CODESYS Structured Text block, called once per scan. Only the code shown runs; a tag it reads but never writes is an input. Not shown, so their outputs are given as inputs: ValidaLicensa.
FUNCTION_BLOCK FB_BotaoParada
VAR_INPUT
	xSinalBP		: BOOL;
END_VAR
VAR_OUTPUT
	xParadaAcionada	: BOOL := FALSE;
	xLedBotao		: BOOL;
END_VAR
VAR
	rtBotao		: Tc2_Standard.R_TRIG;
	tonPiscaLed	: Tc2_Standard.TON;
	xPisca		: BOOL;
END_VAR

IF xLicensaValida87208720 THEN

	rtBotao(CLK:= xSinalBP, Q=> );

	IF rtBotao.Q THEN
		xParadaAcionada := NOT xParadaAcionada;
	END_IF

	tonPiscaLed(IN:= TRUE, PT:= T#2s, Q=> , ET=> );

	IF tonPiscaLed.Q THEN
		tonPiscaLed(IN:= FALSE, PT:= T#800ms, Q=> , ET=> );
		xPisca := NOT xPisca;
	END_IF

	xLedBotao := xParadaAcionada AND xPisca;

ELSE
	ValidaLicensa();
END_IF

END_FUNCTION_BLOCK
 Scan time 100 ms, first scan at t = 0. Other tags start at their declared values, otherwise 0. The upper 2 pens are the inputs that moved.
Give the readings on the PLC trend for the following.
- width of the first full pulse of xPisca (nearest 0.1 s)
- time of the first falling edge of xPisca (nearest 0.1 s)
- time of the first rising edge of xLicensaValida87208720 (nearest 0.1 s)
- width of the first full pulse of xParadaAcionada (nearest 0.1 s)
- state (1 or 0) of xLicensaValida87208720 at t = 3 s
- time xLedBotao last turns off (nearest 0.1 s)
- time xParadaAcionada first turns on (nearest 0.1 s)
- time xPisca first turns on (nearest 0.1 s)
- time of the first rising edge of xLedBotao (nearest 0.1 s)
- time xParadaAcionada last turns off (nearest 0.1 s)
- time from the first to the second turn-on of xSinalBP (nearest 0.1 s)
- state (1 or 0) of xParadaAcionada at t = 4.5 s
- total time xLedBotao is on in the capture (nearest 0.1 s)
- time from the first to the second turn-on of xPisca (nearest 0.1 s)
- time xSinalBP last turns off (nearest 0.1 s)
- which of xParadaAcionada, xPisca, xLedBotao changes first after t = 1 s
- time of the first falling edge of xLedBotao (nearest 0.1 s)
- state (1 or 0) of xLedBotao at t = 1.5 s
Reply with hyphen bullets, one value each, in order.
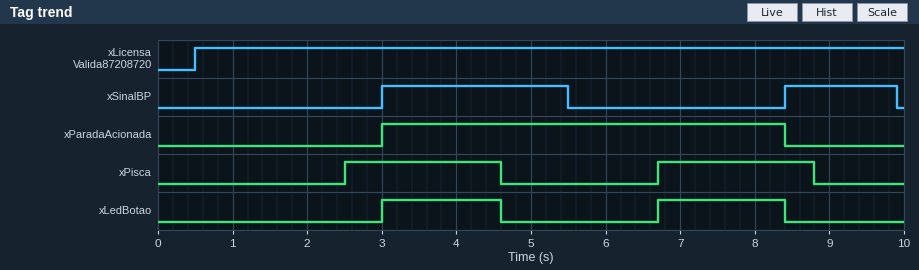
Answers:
- 2.1 s
- 4.6 s
- 0.5 s
- 5.4 s
- 1
- 8.4 s
- 3.0 s
- 2.5 s
- 3.0 s
- 8.4 s
- 5.4 s
- 1
- 3.3 s
- 4.2 s
- 9.9 s
- xPisca
- 4.6 s
- 0
